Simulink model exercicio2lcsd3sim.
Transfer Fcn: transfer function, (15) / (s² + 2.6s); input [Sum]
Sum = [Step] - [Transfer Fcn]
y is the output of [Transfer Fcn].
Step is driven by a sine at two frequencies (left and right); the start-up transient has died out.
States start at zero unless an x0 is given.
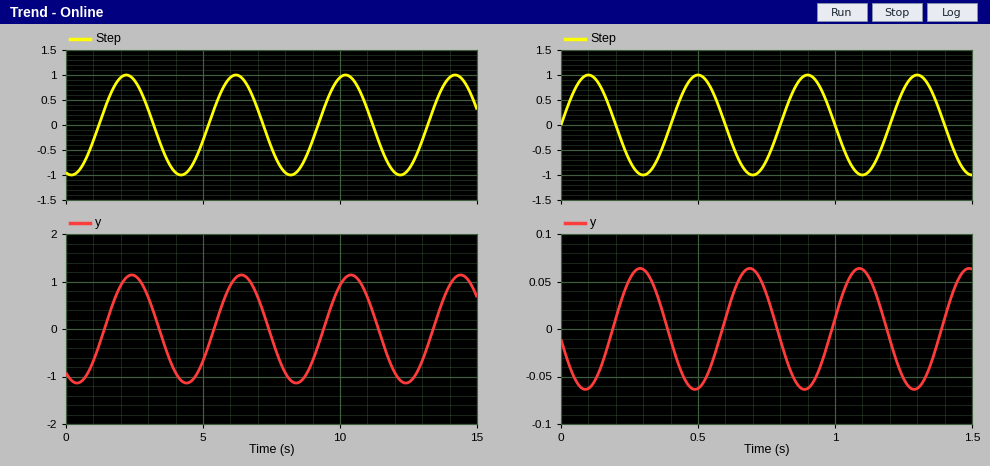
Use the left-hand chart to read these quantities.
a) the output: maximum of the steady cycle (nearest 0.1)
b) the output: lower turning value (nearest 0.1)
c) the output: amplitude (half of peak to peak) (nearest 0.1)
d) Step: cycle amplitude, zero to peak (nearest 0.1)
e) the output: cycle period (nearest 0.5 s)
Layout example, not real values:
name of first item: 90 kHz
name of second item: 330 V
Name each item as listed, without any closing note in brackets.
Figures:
the output: maximum of the steady cycle: 1.1
the output: lower turning value: -1.1
the output: amplitude (half of peak to peak): 1.1
Step: cycle amplitude, zero to peak: 1.0
the output: cycle period: 4.0 s
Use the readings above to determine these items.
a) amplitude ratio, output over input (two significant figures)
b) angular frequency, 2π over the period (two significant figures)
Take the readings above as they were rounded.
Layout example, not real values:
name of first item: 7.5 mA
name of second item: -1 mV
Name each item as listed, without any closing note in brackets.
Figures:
amplitude ratio, output over input: 1.1
angular frequency, 2π over the period: 1.6 rad/s
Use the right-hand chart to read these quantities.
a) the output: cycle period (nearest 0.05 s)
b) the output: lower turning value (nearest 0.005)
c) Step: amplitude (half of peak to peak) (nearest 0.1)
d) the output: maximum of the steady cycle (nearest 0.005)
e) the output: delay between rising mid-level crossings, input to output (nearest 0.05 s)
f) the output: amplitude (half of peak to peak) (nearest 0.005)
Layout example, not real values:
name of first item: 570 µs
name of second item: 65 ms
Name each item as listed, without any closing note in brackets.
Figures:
the output: cycle period: 0.40 s
the output: lower turning value: -0.065
Step: amplitude (half of peak to peak): 1.0
the output: maximum of the steady cycle: 0.065
the output: delay between rising mid-level crossings, input to output: 0.20 s
the output: amplitude (half of peak to peak): 0.065
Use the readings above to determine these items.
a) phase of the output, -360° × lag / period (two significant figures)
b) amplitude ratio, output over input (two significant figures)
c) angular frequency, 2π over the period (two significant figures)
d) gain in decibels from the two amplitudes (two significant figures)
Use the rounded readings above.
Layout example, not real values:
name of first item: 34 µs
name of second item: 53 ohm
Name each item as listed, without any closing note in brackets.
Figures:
phase of the output, -360° × lag / period: -180°
amplitude ratio, output over input: 0.065
angular frequency, 2π over the period: 16 rad/s
gain in decibels from the two amplitudes: -24 dB
